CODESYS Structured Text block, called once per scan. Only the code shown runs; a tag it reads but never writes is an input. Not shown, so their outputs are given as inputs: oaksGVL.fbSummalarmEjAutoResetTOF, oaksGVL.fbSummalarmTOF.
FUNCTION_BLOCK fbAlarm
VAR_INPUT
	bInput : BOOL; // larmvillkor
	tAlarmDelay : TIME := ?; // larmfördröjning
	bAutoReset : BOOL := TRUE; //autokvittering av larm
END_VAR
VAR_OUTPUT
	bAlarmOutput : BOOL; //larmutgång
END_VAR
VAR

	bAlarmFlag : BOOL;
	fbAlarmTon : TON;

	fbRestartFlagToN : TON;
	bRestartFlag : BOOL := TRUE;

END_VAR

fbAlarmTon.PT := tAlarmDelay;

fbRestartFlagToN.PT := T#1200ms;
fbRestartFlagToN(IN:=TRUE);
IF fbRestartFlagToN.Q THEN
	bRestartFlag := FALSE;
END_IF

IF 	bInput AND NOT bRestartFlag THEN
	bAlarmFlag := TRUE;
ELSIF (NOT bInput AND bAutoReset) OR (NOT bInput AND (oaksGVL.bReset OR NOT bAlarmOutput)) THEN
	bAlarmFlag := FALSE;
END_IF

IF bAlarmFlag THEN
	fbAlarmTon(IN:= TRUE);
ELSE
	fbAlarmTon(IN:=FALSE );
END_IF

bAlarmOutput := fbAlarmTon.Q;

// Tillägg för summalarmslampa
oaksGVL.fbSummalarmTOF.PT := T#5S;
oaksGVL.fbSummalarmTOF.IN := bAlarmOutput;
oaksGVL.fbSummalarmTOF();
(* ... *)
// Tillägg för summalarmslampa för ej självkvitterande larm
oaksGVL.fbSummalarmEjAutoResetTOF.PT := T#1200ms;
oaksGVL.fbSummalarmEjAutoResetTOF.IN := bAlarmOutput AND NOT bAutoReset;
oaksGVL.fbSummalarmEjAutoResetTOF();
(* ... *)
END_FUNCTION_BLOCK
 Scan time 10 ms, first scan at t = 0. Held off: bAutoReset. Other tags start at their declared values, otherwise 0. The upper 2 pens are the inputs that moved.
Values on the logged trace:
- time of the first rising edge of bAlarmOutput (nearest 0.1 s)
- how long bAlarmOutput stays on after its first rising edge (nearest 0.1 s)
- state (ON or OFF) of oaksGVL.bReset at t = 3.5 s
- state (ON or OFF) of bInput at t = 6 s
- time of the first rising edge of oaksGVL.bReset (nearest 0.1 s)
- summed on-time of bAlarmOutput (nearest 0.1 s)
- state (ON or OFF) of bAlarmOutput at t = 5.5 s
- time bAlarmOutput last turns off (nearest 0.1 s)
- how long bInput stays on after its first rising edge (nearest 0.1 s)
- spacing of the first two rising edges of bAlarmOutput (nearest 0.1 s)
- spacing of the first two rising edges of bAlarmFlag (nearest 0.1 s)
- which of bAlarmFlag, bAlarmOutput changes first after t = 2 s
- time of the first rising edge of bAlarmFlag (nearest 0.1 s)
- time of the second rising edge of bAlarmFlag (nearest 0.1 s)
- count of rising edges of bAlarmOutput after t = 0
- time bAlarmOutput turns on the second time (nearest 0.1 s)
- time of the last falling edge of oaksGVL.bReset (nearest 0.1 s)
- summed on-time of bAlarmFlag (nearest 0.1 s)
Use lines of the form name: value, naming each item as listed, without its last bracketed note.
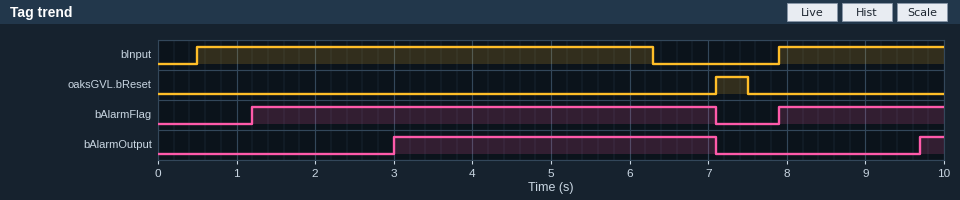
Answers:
time of the first rising edge of bAlarmOutput: 3.0 s
how long bAlarmOutput stays on after its first rising edge: 4.1 s
state (ON or OFF) of oaksGVL.bReset at t = 3.5 s: OFF
state (ON or OFF) of bInput at t = 6 s: ON
time of the first rising edge of oaksGVL.bReset: 7.1 s
summed on-time of bAlarmOutput: 4.4 s
state (ON or OFF) of bAlarmOutput at t = 5.5 s: ON
time bAlarmOutput last turns off: 7.1 s
how long bInput stays on after its first rising edge: 5.8 s
spacing of the first two rising edges of bAlarmOutput: 6.7 s
spacing of the first two rising edges of bAlarmFlag: 6.7 s
which of bAlarmFlag, bAlarmOutput changes first after t = 2 s: bAlarmOutput
time of the first rising edge of bAlarmFlag: 1.2 s
time of the second rising edge of bAlarmFlag: 7.9 s
count of rising edges of bAlarmOutput after t = 0: 2
time bAlarmOutput turns on the second time: 9.7 s
time of the last falling edge of oaksGVL.bReset: 7.5 s
summed on-time of bAlarmFlag: 8.0 s
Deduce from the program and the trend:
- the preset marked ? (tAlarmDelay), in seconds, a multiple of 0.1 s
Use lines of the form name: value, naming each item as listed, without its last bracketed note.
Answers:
the preset marked ? (tAlarmDelay), in seconds, a multiple of 0.1 s: 1.8 s
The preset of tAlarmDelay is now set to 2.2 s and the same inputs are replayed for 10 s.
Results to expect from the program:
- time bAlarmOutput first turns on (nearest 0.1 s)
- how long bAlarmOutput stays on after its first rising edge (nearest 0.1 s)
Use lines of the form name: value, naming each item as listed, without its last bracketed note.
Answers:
time bAlarmOutput first turns on: 3.4 s
how long bAlarmOutput stays on after its first rising edge: 3.7 s
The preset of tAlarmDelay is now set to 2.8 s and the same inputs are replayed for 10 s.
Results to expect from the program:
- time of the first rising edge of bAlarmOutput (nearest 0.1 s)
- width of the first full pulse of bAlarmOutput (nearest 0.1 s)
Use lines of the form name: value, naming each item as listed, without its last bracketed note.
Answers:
time of the first rising edge of bAlarmOutput: 4.0 s
width of the first full pulse of bAlarmOutput: 3.1 s
